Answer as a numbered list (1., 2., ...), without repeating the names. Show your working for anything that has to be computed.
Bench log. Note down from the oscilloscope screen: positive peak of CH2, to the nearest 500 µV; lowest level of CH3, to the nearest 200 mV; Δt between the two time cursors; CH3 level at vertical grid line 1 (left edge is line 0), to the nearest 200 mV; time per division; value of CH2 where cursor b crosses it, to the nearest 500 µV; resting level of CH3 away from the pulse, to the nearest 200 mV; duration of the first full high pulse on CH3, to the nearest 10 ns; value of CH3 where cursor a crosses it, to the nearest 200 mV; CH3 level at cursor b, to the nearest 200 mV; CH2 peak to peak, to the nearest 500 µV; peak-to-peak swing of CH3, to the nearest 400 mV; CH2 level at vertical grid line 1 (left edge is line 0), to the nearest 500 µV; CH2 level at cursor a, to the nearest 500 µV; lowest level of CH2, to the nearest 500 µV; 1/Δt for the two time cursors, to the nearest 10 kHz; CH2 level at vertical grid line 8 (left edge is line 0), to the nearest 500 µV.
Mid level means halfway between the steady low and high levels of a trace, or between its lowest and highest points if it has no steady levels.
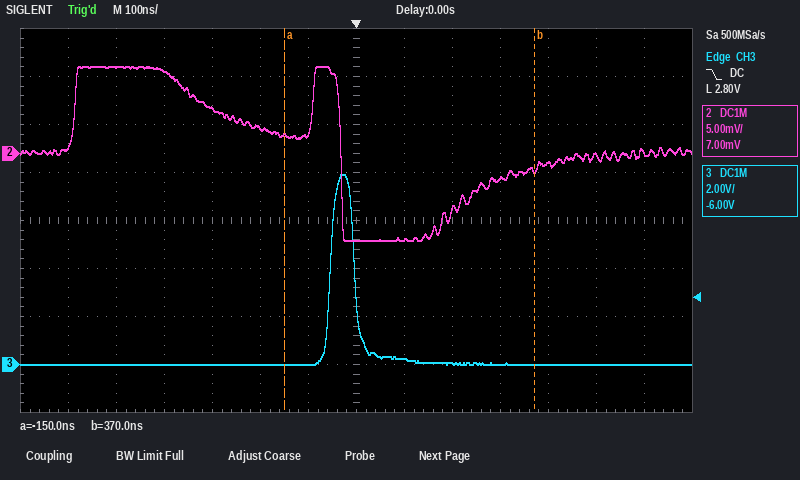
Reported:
1. 9.0 mV
2. 0.0 V
3. 370 ns − (-150 ns) = 520 ns
4. 0.0 V
5. 100 ns
6. -1.5 mV
7. 0.0 V
8. 50 ns
9. 0.0 V
10. 0.0 V
11. 9.0 mV − (-9.0 mV) = 18.0 mV
12. 8.0 V
13. 500 µV
14. 2.0 mV
15. -9.0 mV
16. 1 / 520 ns ≈ 1.92 MHz
17. -9.0 mV
